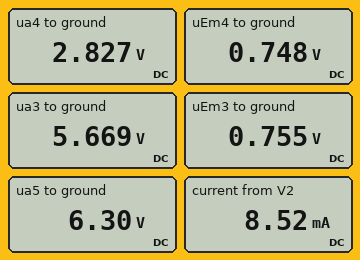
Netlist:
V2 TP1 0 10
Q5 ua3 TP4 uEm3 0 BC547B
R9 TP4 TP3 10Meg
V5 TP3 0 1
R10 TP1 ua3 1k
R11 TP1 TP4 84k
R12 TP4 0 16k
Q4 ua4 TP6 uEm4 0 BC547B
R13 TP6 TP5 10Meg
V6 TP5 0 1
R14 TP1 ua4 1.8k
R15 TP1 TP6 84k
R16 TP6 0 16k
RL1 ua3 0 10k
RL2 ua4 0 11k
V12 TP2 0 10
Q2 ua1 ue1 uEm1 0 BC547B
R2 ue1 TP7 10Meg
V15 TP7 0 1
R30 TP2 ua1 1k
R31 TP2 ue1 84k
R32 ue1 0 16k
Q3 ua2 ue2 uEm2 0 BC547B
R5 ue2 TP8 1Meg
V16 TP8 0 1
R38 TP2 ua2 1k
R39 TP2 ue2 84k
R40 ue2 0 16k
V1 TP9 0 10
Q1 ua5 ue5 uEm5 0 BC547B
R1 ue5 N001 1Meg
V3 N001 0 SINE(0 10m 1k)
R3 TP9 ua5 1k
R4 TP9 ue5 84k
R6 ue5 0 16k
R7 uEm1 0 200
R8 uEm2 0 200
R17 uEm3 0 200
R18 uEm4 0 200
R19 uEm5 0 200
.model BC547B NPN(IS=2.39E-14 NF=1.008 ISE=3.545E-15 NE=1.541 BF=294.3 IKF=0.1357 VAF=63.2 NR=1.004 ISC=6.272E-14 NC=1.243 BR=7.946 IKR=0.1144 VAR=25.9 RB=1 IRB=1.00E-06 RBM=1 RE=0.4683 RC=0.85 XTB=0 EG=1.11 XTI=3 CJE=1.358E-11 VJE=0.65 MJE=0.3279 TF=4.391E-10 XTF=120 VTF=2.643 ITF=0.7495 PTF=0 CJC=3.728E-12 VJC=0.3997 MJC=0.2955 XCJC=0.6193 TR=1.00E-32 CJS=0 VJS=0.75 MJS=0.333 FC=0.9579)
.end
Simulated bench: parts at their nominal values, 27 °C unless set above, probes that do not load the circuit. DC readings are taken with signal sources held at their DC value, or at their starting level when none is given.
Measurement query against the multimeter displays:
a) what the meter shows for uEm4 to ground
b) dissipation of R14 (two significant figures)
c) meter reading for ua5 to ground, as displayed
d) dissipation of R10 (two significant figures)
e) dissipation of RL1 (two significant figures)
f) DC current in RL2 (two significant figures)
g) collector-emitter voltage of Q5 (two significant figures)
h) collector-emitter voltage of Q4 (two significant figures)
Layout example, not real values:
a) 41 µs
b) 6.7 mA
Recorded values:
a) 0.748 V
b) 29 mW
c) 6.30 V
d) 19 mW
e) 3.2 mW
f) 260 µA
g) 4.9 V
h) 2.1 V
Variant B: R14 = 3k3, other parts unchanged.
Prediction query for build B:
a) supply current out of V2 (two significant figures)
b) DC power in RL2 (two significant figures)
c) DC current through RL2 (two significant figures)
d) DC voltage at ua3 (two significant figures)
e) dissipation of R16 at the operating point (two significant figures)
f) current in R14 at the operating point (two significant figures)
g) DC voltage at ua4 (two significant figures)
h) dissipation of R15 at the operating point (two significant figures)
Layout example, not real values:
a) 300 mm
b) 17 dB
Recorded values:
a) 7.4 mA
b) 39 µW
c) 59 µA
d) 5.7 V
e) 94 µW
f) 2.8 mA
g) 650 mV
h) 920 µW
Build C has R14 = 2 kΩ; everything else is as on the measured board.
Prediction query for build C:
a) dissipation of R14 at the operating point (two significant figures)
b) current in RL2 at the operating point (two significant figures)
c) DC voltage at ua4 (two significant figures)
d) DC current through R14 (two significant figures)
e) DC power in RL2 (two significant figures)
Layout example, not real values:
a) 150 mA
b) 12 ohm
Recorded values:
a) 31 mW
b) 200 µA
c) 2.2 V
d) 3.9 mA
e) 430 µW
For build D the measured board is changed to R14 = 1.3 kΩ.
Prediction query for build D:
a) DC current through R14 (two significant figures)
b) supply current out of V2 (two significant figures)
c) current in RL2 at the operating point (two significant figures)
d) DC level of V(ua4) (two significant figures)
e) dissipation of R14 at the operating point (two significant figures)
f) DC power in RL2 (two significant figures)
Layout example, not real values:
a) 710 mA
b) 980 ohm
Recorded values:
a) 4.2 mA
b) 8.7 mA
c) 420 µA
d) 4.6 V
e) 23 mW
f) 1.9 mW
